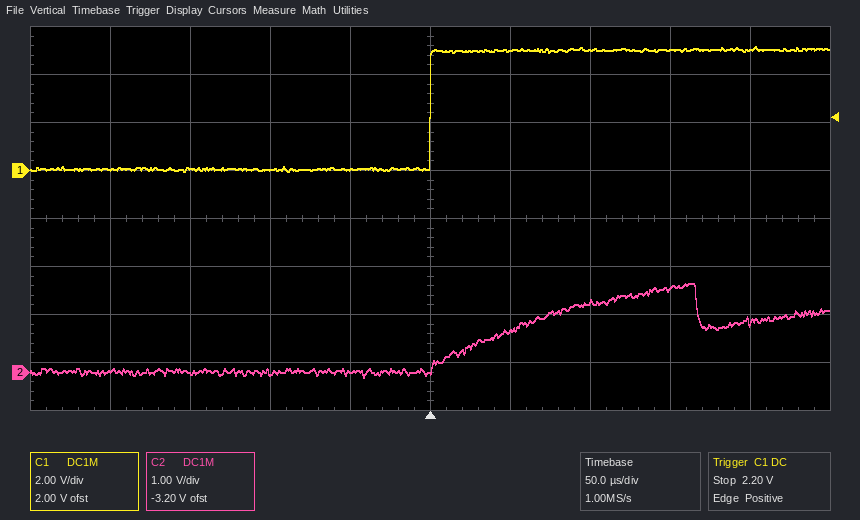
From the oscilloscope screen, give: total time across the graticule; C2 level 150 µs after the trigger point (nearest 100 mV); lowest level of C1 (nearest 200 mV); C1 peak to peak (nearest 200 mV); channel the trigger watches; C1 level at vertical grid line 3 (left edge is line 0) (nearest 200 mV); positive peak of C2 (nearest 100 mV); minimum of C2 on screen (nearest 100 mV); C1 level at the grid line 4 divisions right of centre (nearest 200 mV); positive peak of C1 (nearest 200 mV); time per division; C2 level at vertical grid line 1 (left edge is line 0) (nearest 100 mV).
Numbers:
500 µs
1.7 V
0.0 V
5.2 V
C1
0.0 V
1.8 V
-100 mV
5.0 V
5.2 V
50 µs
0.0 V
